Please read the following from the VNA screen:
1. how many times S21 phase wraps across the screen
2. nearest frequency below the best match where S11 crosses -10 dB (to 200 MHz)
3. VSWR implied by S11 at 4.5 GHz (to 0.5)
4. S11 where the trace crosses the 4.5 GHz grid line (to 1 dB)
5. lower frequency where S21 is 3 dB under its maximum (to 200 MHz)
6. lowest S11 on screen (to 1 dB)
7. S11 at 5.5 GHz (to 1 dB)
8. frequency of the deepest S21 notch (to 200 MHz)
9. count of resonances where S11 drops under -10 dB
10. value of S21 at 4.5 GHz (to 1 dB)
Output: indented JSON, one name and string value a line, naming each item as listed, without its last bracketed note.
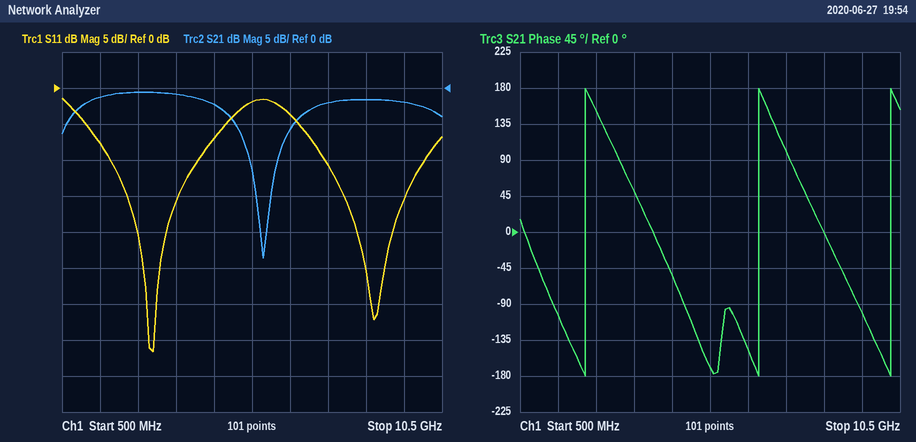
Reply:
{
  "how many times S21 phase wraps across the screen": "3",
  "nearest frequency below the best match where S11 crosses -10 dB": "1.8 GHz",
  "VSWR implied by S11 at 4.5 GHz": "2.5",
  "S11 where the trace crosses the 4.5 GHz grid line": "-7 dB",
  "lower frequency where S21 is 3 dB under its maximum": "800 MHz",
  "lowest S11 on screen": "-37 dB",
  "S11 at 5.5 GHz": "-2 dB",
  "frequency of the deepest S21 notch": "5.8 GHz",
  "count of resonances where S11 drops under -10 dB": "2",
  "value of S21 at 4.5 GHz": "-2 dB"
}
